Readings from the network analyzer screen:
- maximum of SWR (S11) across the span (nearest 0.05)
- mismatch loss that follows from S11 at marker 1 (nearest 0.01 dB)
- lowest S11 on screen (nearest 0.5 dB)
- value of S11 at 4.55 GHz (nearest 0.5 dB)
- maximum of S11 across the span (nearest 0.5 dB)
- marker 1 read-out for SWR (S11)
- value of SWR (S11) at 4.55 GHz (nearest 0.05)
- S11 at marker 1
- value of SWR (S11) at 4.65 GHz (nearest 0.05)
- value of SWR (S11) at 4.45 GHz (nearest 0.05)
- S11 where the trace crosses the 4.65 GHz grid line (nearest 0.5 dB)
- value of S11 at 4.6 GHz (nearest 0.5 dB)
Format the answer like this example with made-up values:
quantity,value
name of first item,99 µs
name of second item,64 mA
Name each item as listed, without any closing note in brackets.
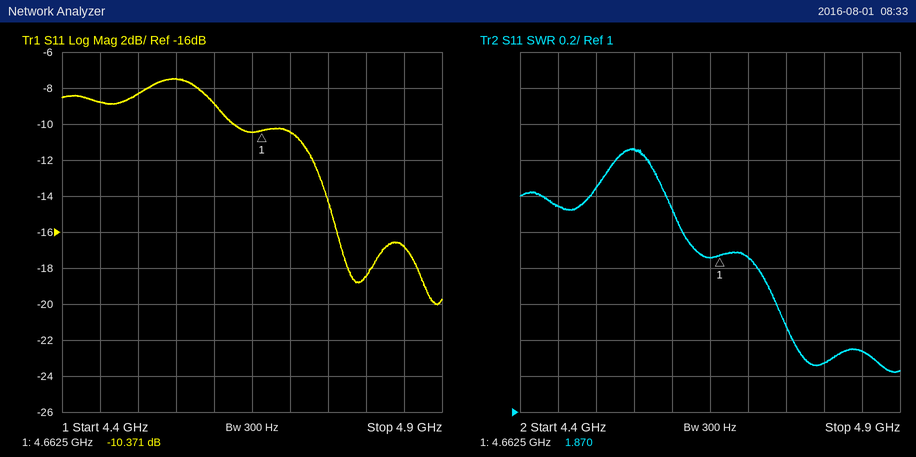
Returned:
quantity,value
maximum of SWR (S11) across the span,2.45
mismatch loss that follows from S11 at marker 1,0.42 dB
lowest S11 on screen,-20.0 dB
value of S11 at 4.55 GHz,-7.5 dB
maximum of S11 across the span,-7.5 dB
marker 1 read-out for SWR,1.870
value of SWR (S11) at 4.55 GHz,2.45
S11 at marker 1,-10.371 dB
value of SWR (S11) at 4.65 GHz,1.85
value of SWR (S11) at 4.45 GHz,2.15
S11 where the trace crosses the 4.65 GHz grid line,-10.5 dB
value of S11 at 4.6 GHz,-9.0 dB
